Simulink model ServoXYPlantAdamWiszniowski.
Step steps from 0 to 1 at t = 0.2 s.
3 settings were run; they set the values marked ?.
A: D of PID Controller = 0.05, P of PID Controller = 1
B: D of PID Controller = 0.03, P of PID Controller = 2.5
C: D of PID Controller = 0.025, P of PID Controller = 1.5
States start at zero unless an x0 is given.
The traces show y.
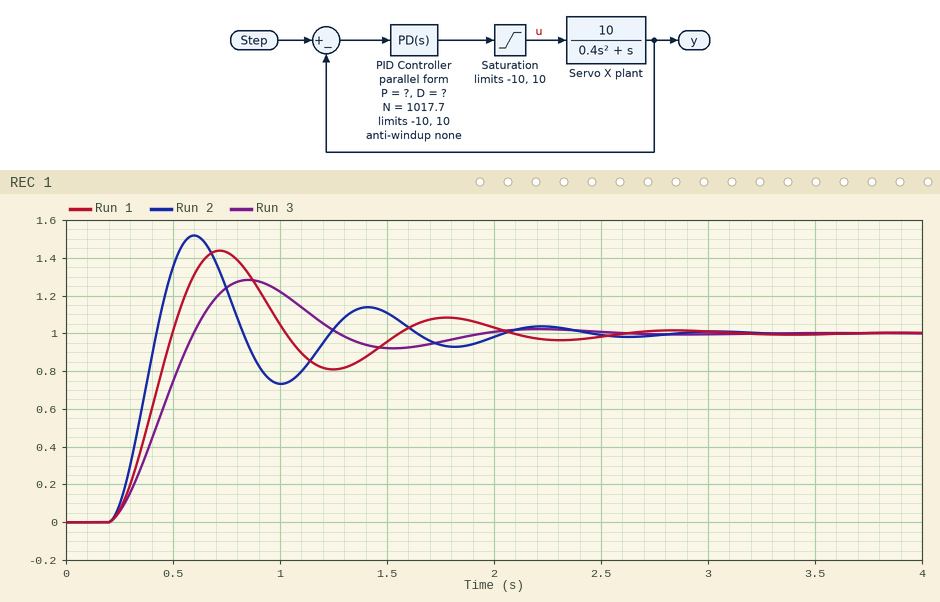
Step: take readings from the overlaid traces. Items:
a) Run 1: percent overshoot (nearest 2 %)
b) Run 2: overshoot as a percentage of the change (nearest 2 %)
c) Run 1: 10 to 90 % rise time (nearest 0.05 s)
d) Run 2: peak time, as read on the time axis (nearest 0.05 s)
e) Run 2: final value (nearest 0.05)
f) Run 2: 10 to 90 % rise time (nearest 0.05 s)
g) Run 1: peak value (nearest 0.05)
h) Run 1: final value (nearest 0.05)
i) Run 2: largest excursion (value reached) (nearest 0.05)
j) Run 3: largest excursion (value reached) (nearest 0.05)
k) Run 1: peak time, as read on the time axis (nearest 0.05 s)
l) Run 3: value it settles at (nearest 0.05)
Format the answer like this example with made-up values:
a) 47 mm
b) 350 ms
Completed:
a) 44 %
b) 52 %
c) 0.20 s
d) 0.60 s
e) 1.00
f) 0.15 s
g) 1.45
h) 1.00
i) 1.50
j) 1.30
k) 0.70 s
l) 1.00
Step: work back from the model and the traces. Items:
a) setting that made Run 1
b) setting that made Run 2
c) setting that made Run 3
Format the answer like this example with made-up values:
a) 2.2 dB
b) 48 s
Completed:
a) C
b) B
c) A
